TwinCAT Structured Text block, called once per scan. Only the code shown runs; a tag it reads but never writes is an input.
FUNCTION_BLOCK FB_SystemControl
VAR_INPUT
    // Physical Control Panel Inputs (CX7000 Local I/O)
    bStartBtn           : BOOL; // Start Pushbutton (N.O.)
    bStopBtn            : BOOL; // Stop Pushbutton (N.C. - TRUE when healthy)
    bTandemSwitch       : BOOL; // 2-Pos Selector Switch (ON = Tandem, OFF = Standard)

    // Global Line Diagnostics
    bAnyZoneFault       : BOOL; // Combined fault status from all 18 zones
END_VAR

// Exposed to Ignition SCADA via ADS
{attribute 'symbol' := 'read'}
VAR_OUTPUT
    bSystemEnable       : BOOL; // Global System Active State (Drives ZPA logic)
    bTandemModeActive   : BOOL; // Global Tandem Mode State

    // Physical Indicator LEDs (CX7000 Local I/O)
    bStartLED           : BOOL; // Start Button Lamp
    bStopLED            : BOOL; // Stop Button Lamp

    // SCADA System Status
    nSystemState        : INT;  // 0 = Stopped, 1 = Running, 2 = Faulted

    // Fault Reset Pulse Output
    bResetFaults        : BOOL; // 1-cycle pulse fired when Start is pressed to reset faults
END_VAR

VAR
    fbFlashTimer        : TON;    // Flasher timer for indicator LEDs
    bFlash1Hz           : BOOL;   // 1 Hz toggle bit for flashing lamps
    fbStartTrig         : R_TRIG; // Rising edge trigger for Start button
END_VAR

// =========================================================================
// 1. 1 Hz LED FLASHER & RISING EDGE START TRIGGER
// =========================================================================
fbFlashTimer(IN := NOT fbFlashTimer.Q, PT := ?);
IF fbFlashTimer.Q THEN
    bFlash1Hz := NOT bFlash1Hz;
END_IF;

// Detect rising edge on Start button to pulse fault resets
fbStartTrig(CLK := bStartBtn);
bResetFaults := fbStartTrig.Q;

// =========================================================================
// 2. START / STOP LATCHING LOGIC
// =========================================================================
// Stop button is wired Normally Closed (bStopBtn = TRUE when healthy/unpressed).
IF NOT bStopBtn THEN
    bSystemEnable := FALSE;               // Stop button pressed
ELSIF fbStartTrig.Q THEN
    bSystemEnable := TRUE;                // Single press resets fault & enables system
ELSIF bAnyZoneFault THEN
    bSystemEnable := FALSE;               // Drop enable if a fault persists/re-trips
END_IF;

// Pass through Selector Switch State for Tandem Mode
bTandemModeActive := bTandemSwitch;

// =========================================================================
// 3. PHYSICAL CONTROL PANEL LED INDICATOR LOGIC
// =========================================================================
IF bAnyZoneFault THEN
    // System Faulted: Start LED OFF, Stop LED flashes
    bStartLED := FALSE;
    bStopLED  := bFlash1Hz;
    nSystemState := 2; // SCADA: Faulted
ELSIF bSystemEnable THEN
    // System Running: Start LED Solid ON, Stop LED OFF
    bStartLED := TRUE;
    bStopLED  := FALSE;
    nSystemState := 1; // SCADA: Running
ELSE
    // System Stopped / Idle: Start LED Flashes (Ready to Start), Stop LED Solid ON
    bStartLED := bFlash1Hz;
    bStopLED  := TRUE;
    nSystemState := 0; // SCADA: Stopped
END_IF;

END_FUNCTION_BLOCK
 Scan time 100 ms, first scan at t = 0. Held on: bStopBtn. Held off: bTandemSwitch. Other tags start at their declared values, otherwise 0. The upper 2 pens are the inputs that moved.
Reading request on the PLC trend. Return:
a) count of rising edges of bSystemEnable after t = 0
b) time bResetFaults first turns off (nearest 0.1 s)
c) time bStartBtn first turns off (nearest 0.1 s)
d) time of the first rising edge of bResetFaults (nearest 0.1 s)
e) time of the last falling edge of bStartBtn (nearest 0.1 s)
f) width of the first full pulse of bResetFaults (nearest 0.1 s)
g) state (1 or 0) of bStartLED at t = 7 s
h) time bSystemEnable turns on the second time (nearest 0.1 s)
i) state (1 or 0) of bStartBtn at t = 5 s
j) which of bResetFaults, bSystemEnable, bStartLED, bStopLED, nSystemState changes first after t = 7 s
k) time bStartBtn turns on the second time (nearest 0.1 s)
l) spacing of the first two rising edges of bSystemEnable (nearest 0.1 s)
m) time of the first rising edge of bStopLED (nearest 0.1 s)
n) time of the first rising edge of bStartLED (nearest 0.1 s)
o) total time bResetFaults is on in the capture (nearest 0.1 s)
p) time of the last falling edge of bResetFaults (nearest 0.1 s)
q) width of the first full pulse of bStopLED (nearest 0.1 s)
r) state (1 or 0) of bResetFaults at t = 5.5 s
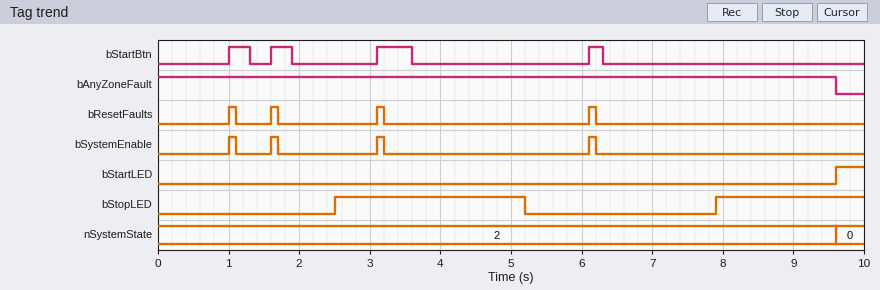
4
1.1 s
1.3 s
1.0 s
6.3 s
0.1 s
0
1.6 s
0
bStopLED
1.6 s
0.6 s
2.5 s
9.6 s
0.4 s
6.2 s
2.7 s
0
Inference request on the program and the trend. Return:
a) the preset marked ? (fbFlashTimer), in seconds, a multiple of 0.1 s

2.5 s
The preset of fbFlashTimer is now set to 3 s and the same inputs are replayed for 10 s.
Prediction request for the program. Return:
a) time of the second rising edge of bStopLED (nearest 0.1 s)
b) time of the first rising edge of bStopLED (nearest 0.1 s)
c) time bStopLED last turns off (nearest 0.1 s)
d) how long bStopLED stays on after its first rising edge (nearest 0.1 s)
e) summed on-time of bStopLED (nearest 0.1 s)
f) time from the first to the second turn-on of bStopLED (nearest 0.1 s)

9.4 s
3.0 s
6.2 s
3.2 s
3.8 s
6.4 s
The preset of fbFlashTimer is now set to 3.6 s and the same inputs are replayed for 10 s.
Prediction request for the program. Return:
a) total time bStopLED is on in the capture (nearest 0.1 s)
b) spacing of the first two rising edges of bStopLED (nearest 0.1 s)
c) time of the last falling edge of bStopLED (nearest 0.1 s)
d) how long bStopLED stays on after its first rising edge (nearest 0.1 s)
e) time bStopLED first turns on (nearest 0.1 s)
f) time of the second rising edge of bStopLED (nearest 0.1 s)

4.2 s
6.0 s
7.4 s
3.8 s
3.6 s
9.6 s
